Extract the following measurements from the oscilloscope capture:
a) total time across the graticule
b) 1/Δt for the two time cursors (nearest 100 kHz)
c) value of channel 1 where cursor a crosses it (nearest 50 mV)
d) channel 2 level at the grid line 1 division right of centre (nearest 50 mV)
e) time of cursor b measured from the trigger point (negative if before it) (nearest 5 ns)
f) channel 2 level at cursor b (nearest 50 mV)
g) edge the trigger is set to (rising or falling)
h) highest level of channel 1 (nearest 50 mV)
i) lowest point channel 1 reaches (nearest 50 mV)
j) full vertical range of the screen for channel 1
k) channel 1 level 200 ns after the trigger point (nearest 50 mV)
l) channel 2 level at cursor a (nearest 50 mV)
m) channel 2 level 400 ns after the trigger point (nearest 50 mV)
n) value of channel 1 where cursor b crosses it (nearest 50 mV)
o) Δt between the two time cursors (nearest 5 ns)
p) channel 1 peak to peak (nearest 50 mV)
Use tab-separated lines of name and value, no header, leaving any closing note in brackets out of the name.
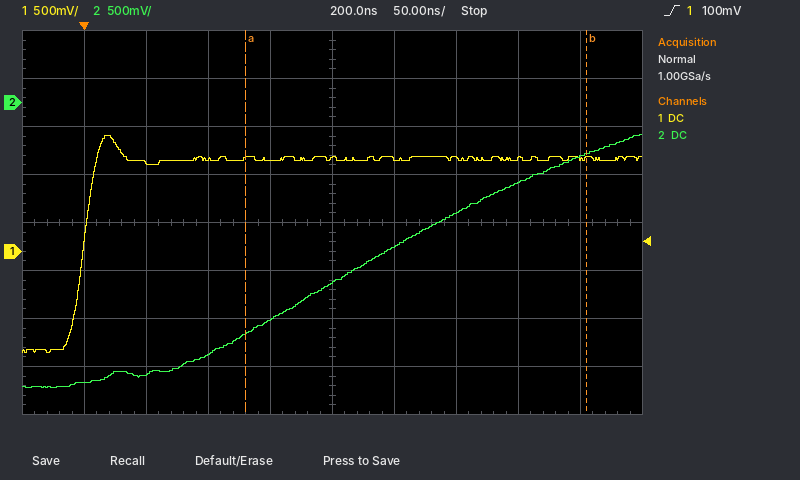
total time across the graticule	500 ns
1/Δt for the two time cursors	3.6 MHz
value of channel 1 where cursor a crosses it	950 mV
channel 2 level at the grid line 1 division right of centre	-1.50 V
time of cursor b measured from the trigger point (negative if before it)	+405 ns
channel 2 level at cursor b	-550 mV
edge the trigger is set to	rising
highest level of channel 1	1.20 V
lowest point channel 1 reaches	-1.05 V
full vertical range of the screen for channel 1	4 V
channel 1 level 200 ns after the trigger point	950 mV
channel 2 level at cursor a	-2.40 V
channel 2 level 400 ns after the trigger point	-550 mV
value of channel 1 where cursor b crosses it	950 mV
Δt between the two time cursors	275 ns
channel 1 peak to peak	2.25 V
